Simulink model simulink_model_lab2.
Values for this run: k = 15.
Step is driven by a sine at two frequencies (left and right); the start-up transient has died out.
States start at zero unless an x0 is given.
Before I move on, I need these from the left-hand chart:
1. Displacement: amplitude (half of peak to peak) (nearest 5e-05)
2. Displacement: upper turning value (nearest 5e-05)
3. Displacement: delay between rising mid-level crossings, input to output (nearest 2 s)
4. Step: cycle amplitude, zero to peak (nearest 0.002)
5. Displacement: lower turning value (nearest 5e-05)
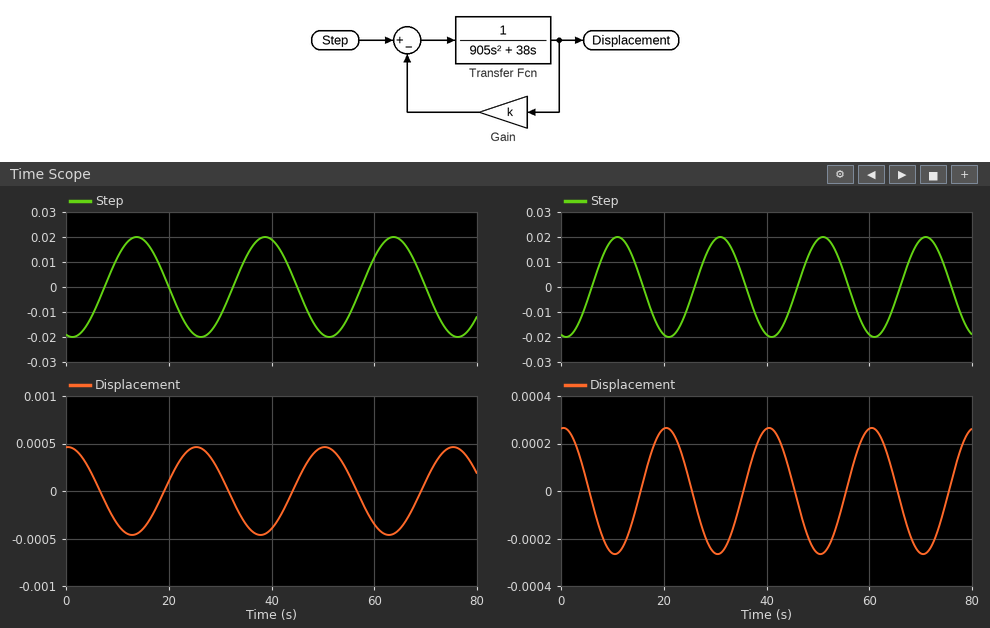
0.00045
0.00045
12 s
0.020
-0.00045
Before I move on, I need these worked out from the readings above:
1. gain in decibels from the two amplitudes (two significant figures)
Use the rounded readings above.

-33 dB
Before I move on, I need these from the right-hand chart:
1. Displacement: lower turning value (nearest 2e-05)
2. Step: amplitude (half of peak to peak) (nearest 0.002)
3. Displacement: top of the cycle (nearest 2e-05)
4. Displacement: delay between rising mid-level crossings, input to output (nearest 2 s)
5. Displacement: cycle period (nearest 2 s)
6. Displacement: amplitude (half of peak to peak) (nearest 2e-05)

-0.00026
0.020
0.00026
10 s
20 s
0.00026
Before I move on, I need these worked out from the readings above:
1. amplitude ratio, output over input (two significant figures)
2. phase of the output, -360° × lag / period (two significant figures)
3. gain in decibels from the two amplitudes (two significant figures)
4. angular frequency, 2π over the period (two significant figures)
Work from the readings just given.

0.013
-180°
-38 dB
0.31 rad/s
